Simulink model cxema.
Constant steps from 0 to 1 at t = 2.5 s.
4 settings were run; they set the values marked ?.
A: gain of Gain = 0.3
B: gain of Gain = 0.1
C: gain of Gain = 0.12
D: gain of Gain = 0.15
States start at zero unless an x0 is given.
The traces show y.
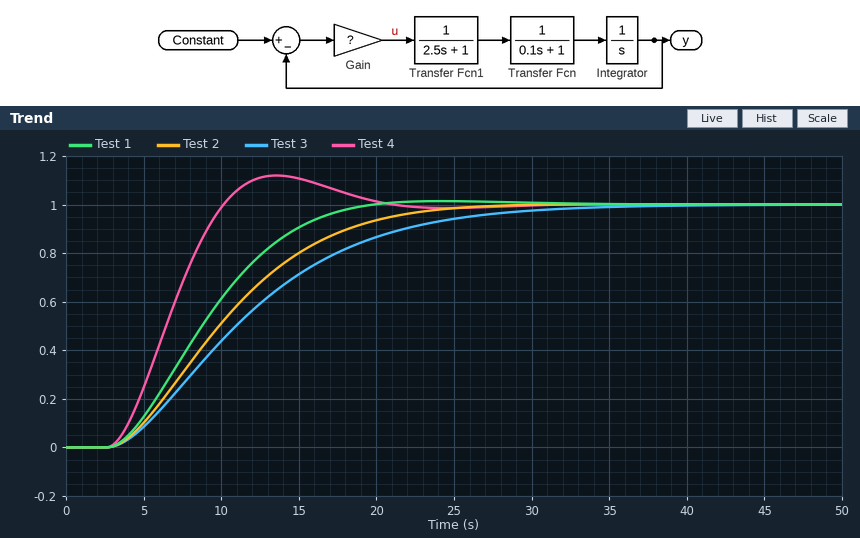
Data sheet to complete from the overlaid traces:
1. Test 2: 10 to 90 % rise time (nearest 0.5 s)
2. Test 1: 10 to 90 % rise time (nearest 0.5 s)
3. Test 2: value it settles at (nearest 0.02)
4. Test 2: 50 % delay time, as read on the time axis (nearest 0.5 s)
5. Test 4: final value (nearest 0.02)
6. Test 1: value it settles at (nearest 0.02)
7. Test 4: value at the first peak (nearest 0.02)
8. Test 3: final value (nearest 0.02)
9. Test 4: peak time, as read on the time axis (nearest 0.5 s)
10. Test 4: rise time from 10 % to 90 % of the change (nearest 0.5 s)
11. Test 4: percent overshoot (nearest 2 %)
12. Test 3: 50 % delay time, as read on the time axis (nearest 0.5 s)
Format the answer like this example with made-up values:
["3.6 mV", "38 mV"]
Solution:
["13.0 s", "10.0 s", "1.00", "10.0 s", "1.00", "1.00", "1.12", "1.00", "13.5 s", "5.0 s", "12 %", "11.0 s"]
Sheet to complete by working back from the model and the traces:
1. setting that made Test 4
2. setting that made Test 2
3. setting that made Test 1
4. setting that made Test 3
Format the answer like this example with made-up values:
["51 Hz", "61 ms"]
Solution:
["A", "C", "D", "B"]
